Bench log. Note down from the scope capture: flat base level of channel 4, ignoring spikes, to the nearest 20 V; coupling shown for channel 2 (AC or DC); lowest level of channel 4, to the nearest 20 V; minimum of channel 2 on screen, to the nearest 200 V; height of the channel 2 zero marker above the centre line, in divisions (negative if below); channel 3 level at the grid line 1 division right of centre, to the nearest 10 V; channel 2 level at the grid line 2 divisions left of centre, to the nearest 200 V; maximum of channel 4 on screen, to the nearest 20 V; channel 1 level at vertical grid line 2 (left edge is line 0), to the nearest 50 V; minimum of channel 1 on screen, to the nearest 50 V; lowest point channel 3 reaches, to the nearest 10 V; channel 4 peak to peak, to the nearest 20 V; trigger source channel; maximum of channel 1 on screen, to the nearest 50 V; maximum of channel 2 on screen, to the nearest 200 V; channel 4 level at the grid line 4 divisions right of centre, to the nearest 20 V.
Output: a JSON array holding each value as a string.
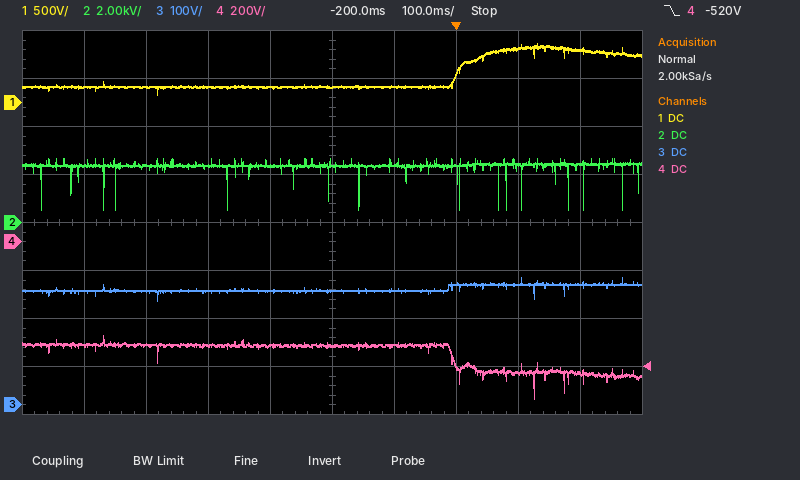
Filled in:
["-540 V", "DC", "-660 V", "600 V", "0.0 div", "240 V", "2.4 kV", "-400 V", "150 V", "100 V", "220 V", "260 V", "channel 4", "600 V", "2.6 kV", "-540 V"]
